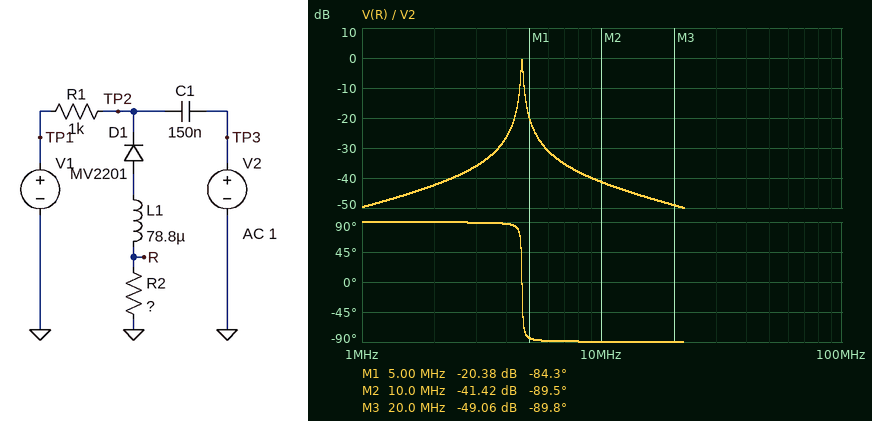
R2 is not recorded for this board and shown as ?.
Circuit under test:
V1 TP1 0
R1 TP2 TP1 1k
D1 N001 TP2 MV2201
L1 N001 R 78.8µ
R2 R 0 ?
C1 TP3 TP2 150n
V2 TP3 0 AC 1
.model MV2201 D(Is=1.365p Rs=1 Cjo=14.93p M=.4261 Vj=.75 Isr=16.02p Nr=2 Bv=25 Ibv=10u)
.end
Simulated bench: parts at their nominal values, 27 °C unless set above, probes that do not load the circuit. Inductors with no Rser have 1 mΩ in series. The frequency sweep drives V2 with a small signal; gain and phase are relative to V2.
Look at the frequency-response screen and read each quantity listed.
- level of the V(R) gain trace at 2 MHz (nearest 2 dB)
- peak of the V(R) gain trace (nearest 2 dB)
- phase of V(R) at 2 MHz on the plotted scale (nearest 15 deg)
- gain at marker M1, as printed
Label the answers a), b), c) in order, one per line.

a) -42 dB
b) 0 dB
c) 90 deg
d) -20.38 dB
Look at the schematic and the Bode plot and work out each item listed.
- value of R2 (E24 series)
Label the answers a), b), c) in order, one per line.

a) 33 Ω
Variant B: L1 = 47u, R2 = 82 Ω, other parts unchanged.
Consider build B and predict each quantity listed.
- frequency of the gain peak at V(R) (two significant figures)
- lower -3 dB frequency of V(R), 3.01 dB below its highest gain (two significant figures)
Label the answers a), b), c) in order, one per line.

a) 6.0 MHz
b) 5.9 MHz
